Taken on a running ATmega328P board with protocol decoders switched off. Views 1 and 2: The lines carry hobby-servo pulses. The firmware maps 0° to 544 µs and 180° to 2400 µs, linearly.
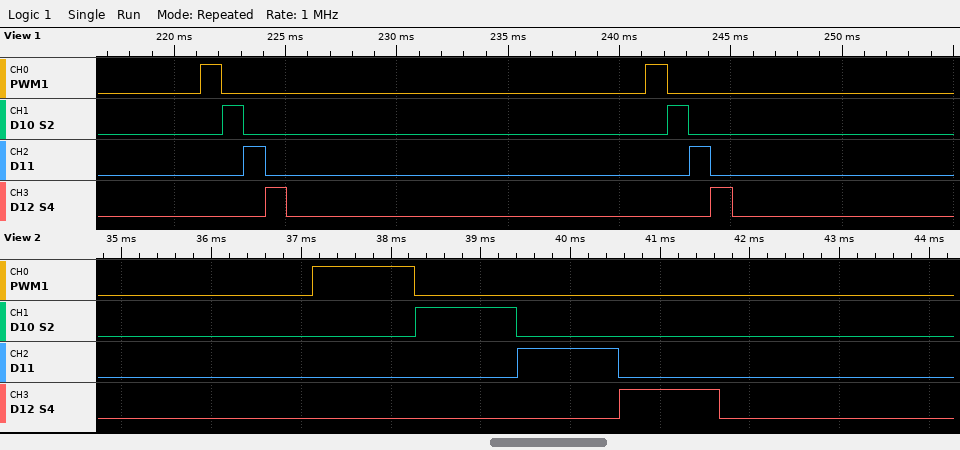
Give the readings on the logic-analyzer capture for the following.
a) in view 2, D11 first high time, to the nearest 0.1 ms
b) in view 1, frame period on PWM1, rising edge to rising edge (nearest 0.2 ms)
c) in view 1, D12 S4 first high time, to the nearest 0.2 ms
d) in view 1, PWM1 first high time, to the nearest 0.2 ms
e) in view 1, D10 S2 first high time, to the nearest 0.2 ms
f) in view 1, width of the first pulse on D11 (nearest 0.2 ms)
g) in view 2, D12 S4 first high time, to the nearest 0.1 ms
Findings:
1.1 ms
20.0 ms
1.0 ms
1.0 ms
1.0 ms
1.0 ms
1.1 ms
